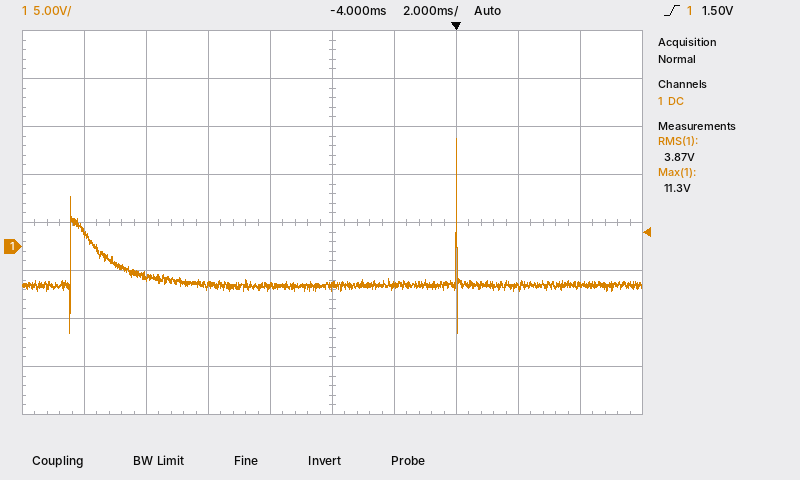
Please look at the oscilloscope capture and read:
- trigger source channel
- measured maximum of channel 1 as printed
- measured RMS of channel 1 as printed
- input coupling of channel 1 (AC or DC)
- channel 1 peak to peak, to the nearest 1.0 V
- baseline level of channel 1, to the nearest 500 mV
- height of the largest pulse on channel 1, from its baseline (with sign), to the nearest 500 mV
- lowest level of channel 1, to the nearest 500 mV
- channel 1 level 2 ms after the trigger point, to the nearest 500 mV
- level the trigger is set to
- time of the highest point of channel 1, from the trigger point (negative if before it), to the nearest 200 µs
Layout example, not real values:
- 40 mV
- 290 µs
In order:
- channel 1
- 11.3 V
- 3.87 V
- DC
- 20.0 V
- -4.0 V
- +15.5 V
- -9.0 V
- -4.0 V
- 1.50 V
- 0.0 ms
